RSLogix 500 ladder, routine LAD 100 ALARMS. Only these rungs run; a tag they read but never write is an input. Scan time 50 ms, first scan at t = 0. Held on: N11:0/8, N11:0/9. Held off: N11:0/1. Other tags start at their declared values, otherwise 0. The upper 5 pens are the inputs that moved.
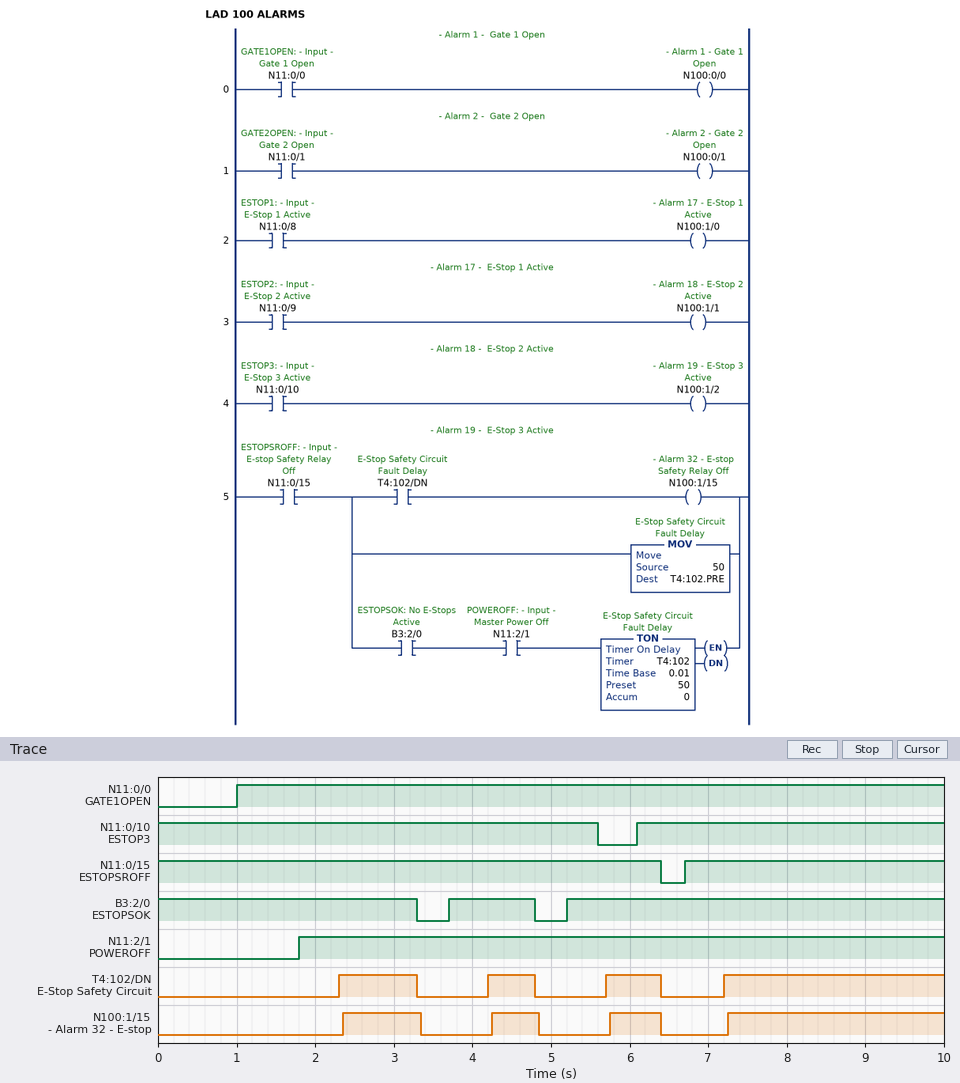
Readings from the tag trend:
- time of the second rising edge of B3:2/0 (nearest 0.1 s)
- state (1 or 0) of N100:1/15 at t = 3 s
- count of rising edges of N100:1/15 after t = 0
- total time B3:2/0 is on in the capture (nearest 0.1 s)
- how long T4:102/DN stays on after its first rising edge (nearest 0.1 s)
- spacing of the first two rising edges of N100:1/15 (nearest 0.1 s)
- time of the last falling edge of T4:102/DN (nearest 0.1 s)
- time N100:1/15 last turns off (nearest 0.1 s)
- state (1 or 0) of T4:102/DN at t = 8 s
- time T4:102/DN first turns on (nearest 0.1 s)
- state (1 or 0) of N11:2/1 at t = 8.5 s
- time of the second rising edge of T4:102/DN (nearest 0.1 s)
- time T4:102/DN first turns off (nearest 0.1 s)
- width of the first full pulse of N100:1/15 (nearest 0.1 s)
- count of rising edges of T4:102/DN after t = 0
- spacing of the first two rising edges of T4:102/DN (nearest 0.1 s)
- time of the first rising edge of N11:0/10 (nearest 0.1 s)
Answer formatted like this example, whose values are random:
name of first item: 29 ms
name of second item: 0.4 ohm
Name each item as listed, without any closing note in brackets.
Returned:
time of the second rising edge of B3:2/0: 5.2 s
state (1 or 0) of N100:1/15 at t = 3 s: 1
count of rising edges of N100:1/15 after t = 0: 4
total time B3:2/0 is on in the capture: 9.2 s
how long T4:102/DN stays on after its first rising edge: 1.0 s
spacing of the first two rising edges of N100:1/15: 1.9 s
time of the last falling edge of T4:102/DN: 6.4 s
time N100:1/15 last turns off: 6.4 s
state (1 or 0) of T4:102/DN at t = 8 s: 1
time T4:102/DN first turns on: 2.3 s
state (1 or 0) of N11:2/1 at t = 8.5 s: 1
time of the second rising edge of T4:102/DN: 4.2 s
time T4:102/DN first turns off: 3.3 s
width of the first full pulse of N100:1/15: 1.0 s
count of rising edges of T4:102/DN after t = 0: 4
spacing of the first two rising edges of T4:102/DN: 1.9 s
time of the first rising edge of N11:0/10: 6.1 s
